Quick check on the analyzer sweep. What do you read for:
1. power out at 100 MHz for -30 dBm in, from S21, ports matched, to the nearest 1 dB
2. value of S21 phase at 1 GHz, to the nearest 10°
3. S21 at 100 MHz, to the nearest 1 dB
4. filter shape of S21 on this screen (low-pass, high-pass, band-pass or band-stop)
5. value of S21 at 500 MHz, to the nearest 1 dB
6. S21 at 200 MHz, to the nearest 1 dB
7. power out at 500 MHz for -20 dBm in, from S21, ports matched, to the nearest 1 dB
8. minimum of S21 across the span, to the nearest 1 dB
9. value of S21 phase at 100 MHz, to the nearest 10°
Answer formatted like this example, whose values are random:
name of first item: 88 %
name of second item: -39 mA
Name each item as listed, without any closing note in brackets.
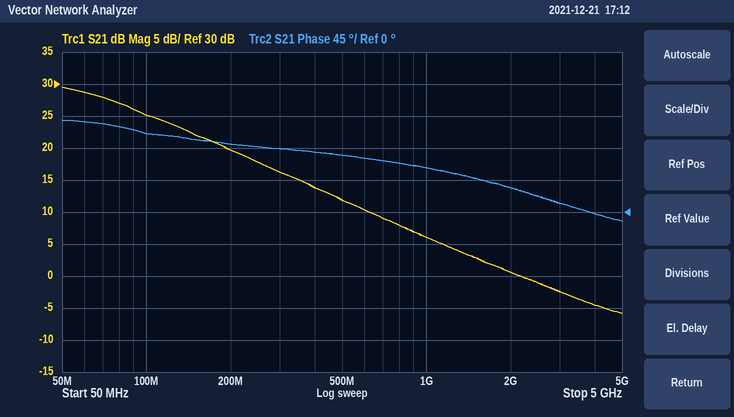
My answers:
power out at 100 MHz for -30 dBm in, from S21, ports matched, to the nearest 1 dB: -5 dBm
value of S21 phase at 1 GHz, to the nearest 10°: 60°
S21 at 100 MHz, to the nearest 1 dB: 25 dB
filter shape of S21 on this screen: low-pass
value of S21 at 500 MHz, to the nearest 1 dB: 12 dB
S21 at 200 MHz, to the nearest 1 dB: 20 dB
power out at 500 MHz for -20 dBm in, from S21, ports matched, to the nearest 1 dB: -8 dBm
minimum of S21 across the span, to the nearest 1 dB: -6 dB
value of S21 phase at 100 MHz, to the nearest 10°: 110°
